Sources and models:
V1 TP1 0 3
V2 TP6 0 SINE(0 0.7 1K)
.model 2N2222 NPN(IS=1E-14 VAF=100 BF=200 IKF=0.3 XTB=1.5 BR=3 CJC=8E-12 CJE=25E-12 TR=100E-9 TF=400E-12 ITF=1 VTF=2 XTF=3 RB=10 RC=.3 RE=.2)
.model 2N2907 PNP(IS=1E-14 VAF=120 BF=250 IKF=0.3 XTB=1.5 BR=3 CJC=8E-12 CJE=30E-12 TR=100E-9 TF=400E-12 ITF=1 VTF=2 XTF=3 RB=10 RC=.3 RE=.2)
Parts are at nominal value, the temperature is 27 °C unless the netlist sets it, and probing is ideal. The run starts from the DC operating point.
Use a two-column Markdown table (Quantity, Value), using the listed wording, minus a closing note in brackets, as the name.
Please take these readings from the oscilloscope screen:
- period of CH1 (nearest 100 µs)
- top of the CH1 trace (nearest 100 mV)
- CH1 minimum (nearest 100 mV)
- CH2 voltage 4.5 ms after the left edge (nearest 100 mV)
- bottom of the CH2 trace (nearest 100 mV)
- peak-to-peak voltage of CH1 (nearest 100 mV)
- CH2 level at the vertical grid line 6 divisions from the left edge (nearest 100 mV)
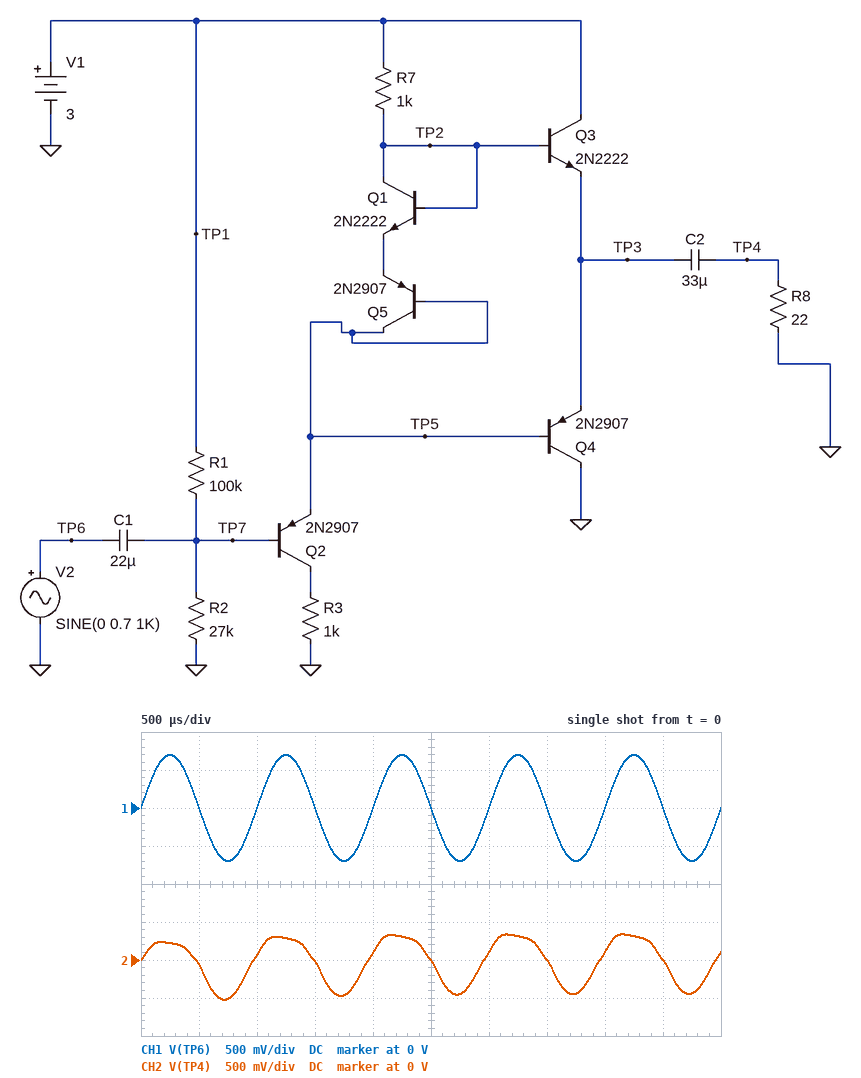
| Quantity | Value |
|---|---|
| period of CH1 | 1.0 ms |
| top of the CH1 trace | 700 mV |
| CH1 minimum | -700 mV |
| CH2 voltage 4.5 ms after the left edge | 0 V |
| bottom of the CH2 trace | -500 mV |
| peak-to-peak voltage of CH1 | 1.4 V |
| CH2 level at the vertical grid line 6 divisions from the left edge | 100 mV |
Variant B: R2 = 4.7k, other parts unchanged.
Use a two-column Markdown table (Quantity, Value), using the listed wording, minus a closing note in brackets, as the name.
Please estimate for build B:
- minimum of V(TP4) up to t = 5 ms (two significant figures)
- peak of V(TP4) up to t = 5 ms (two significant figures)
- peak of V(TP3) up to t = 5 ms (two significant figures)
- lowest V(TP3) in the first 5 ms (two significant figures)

| Quantity | Value |
|---|---|
| minimum of V(TP4) up to t = 5 ms | -560 mV |
| peak of V(TP4) up to t = 5 ms | 480 mV |
| peak of V(TP3) up to t = 5 ms | 2.0 V |
| lowest V(TP3) in the first 5 ms | 990 mV |
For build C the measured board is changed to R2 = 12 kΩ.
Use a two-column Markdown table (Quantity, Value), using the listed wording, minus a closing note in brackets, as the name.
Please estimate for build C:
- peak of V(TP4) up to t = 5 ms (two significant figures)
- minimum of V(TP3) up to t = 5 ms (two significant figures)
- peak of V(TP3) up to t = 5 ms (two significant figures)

| Quantity | Value |
|---|---|
| peak of V(TP4) up to t = 5 ms | 450 mV |
| minimum of V(TP3) up to t = 5 ms | 1.1 V |
| peak of V(TP3) up to t = 5 ms | 2.1 V |
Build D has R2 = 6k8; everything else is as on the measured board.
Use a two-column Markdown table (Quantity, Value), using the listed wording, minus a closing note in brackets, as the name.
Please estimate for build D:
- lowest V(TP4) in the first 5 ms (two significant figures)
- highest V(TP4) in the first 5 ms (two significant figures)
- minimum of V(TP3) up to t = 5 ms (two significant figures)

| Quantity | Value |
|---|---|
| lowest V(TP4) in the first 5 ms | -560 mV |
| highest V(TP4) in the first 5 ms | 470 mV |
| minimum of V(TP3) up to t = 5 ms | 1.0 V |
